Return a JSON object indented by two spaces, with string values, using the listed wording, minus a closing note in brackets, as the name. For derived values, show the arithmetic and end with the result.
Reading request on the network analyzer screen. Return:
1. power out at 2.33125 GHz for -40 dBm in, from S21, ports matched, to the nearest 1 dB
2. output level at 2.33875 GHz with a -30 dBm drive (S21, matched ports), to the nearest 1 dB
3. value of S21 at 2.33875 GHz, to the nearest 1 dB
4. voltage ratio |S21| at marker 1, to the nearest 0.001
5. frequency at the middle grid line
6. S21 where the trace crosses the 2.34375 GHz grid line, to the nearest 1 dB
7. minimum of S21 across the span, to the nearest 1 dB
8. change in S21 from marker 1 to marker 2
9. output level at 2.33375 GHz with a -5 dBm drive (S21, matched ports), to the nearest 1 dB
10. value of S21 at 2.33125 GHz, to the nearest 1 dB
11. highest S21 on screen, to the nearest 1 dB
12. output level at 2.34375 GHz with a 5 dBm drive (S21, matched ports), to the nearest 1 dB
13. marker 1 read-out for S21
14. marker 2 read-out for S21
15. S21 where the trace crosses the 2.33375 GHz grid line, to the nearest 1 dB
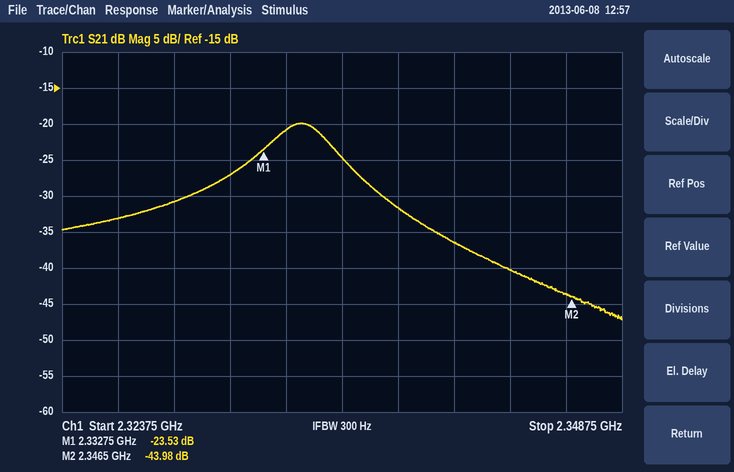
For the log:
{
  "power out at 2.33125 GHz for -40 dBm in, from S21, ports matched, to the nearest 1 dB": "-40 dBm + (-27 dB) = -67 dBm",
  "output level at 2.33875 GHz with a -30 dBm drive (S21, matched ports), to the nearest 1 dB": "-30 dBm + (-32 dB) = -62 dBm",
  "value of S21 at 2.33875 GHz, to the nearest 1 dB": "-32 dB",
  "voltage ratio |S21| at marker 1, to the nearest 0.001": "10^(-23.53/20) ≈ 0.067",
  "frequency at the middle grid line": "2.33625 GHz",
  "S21 where the trace crosses the 2.34375 GHz grid line, to the nearest 1 dB": "-40 dB",
  "minimum of S21 across the span, to the nearest 1 dB": "-47 dB",
  "change in S21 from marker 1 to marker 2": "-43.98 − (-23.53) = -20.45 dB",
  "output level at 2.33375 GHz with a -5 dBm drive (S21, matched ports), to the nearest 1 dB": "-5 dBm + (-21 dB) = -26 dBm",
  "value of S21 at 2.33125 GHz, to the nearest 1 dB": "-27 dB",
  "highest S21 on screen, to the nearest 1 dB": "-20 dB",
  "output level at 2.34375 GHz with a 5 dBm drive (S21, matched ports), to the nearest 1 dB": "5 dBm + (-40 dB) = -35 dBm",
  "marker 1 read-out for S21": "-23.53 dB",
  "marker 2 read-out for S21": "-43.98 dB",
  "S21 where the trace crosses the 2.33375 GHz grid line, to the nearest 1 dB": "-21 dB"
}
